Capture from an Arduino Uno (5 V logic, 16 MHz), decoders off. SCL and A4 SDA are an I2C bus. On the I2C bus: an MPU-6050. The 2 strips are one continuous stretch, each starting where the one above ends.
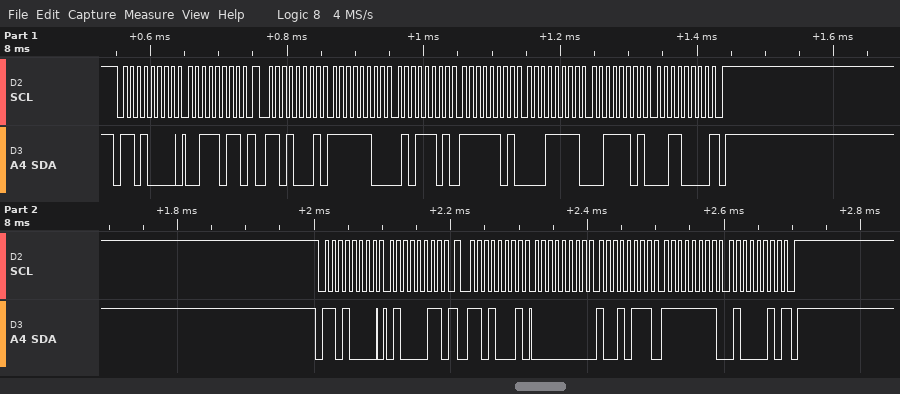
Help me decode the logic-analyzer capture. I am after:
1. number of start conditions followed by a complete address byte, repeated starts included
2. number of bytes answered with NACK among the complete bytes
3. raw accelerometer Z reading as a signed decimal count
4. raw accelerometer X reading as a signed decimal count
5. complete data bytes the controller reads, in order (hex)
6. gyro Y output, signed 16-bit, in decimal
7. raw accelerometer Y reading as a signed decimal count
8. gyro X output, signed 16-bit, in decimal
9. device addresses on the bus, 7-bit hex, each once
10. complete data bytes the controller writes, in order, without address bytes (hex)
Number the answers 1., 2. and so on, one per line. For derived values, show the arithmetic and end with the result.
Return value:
1. 4
2. 2
3. 0x3D30 = 15664
4. 0xFC5D = -931
5. FC 5D FD 1F 3D 30 00 97 FF 42
6. 0xFF42 = -190
7. 0xFD1F = -737
8. 0x0097 = 151
9. 0x68
10. 3B 43
